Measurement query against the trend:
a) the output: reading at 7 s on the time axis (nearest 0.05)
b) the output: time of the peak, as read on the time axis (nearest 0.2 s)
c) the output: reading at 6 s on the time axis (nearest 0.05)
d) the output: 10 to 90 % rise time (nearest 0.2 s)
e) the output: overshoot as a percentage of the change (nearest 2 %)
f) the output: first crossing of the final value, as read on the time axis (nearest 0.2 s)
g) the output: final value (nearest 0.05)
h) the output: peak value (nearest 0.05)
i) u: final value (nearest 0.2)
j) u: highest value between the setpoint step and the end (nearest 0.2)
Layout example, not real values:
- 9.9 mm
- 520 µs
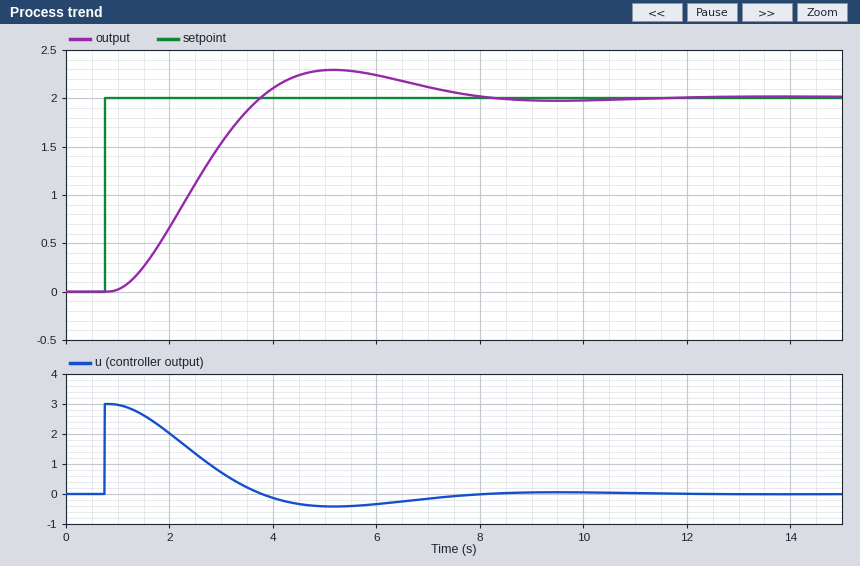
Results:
- 2.10
- 5.2 s
- 2.25
- 2.0 s
- 14 %
- 3.8 s
- 2.00
- 2.30
- 0.0
- 3.0
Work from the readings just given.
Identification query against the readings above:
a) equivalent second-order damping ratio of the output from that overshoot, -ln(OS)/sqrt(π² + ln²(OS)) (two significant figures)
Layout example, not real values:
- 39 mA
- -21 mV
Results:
- 0.53
